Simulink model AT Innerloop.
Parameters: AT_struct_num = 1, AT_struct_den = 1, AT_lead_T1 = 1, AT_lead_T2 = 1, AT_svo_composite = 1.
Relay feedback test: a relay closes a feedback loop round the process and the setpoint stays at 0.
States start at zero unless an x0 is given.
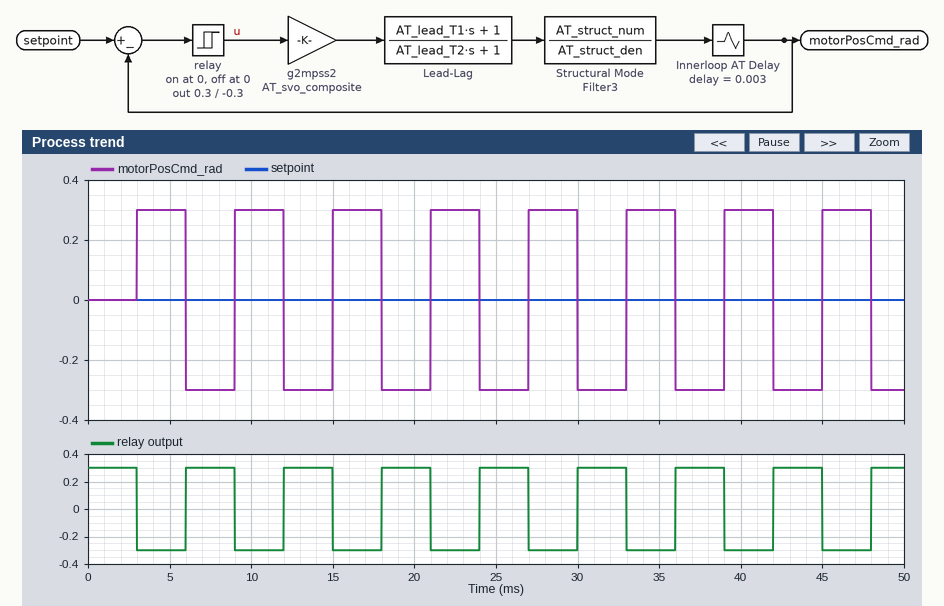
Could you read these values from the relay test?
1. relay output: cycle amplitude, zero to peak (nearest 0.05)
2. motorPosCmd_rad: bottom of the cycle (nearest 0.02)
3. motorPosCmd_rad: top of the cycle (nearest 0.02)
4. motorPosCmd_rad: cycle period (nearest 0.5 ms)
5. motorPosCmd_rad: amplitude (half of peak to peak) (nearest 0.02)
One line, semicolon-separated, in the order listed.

0.30; -0.30; 0.30; 6.0 ms; 0.30
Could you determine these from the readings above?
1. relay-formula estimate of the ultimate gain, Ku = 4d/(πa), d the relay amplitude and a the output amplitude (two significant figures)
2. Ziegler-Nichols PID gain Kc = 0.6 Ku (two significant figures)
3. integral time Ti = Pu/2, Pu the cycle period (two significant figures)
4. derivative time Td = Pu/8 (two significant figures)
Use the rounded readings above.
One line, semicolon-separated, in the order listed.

1.3; 0.78; 3.0 ms; 0.75 ms
